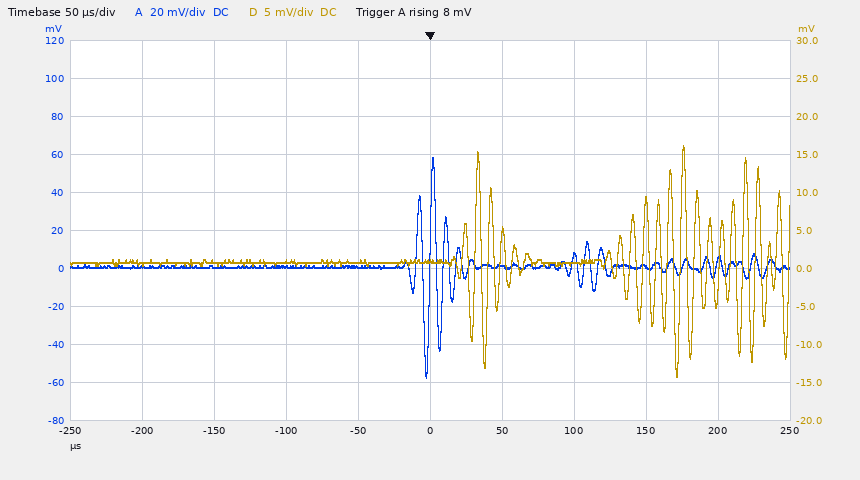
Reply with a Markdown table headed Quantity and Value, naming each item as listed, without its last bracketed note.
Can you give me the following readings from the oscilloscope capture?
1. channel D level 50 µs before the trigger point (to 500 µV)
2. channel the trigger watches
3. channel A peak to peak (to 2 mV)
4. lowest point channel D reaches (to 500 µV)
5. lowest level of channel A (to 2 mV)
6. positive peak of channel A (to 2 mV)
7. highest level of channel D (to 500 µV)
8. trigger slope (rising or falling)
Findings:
| Quantity | Value |
|---|---|
| channel D level 50 µs before the trigger point | 1.0 mV |
| channel the trigger watches | channel A |
| channel A peak to peak | 116 mV |
| lowest point channel D reaches | -14.0 mV |
| lowest level of channel A | -58 mV |
| positive peak of channel A | 58 mV |
| highest level of channel D | 16.0 mV |
| trigger slope | rising |
